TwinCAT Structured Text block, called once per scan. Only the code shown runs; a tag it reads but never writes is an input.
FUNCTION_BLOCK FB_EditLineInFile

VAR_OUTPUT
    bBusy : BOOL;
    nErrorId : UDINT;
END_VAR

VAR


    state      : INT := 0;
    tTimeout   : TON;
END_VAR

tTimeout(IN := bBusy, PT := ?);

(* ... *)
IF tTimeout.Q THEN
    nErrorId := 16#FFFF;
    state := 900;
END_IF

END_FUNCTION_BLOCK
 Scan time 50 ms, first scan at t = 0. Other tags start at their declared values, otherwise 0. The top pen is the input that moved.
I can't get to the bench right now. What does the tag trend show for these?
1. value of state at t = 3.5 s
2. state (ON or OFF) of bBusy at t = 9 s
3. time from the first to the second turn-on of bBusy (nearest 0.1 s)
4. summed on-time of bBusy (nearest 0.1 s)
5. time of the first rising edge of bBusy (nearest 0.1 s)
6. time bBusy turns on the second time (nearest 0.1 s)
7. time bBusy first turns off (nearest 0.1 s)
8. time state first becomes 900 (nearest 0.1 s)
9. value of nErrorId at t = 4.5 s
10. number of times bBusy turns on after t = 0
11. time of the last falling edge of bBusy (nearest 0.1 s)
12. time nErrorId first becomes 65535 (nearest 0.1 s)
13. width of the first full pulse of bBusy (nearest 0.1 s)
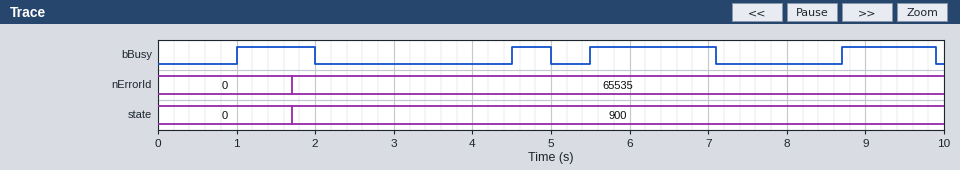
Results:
900
ON
3.5 s
4.3 s
1.0 s
4.5 s
2.0 s
1.7 s
65535
4
9.9 s
1.7 s
1.0 s
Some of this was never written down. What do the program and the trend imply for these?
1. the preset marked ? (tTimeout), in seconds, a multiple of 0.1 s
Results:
0.7 s
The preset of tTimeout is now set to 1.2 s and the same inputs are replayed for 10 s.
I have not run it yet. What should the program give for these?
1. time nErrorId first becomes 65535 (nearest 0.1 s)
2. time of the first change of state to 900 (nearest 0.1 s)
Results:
6.7 s
6.7 s
